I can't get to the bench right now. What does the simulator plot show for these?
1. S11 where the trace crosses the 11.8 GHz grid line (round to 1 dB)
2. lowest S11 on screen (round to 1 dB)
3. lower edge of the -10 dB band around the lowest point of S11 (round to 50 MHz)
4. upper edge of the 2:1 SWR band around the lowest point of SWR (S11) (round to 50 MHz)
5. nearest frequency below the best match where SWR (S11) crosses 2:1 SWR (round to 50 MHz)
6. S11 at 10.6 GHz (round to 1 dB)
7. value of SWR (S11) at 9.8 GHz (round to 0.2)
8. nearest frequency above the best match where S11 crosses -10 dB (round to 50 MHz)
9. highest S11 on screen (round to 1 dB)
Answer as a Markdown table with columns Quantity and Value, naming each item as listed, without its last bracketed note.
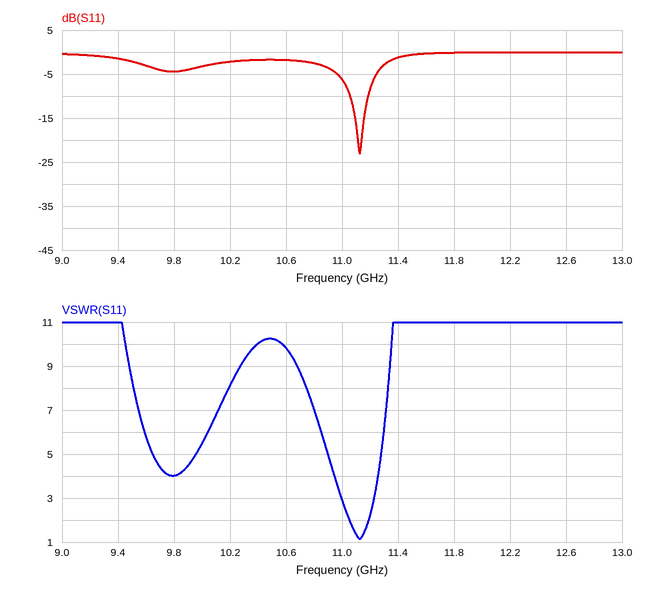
| Quantity | Value |
|---|---|
| S11 where the trace crosses the 11.8 GHz grid line | 0 dB |
| lowest S11 on screen | -23 dB |
| lower edge of the -10 dB band around the lowest point of S11 | 11.05 GHz |
| upper edge of the 2:1 SWR band around the lowest point of SWR (S11) | 11.20 GHz |
| nearest frequency below the best match where SWR (S11) crosses 2:1 SWR | 11.05 GHz |
| S11 at 10.6 GHz | -2 dB |
| value of SWR (S11) at 9.8 GHz | 4.0 |
| nearest frequency above the best match where S11 crosses -10 dB | 11.20 GHz |
| highest S11 on screen | 0 dB |
